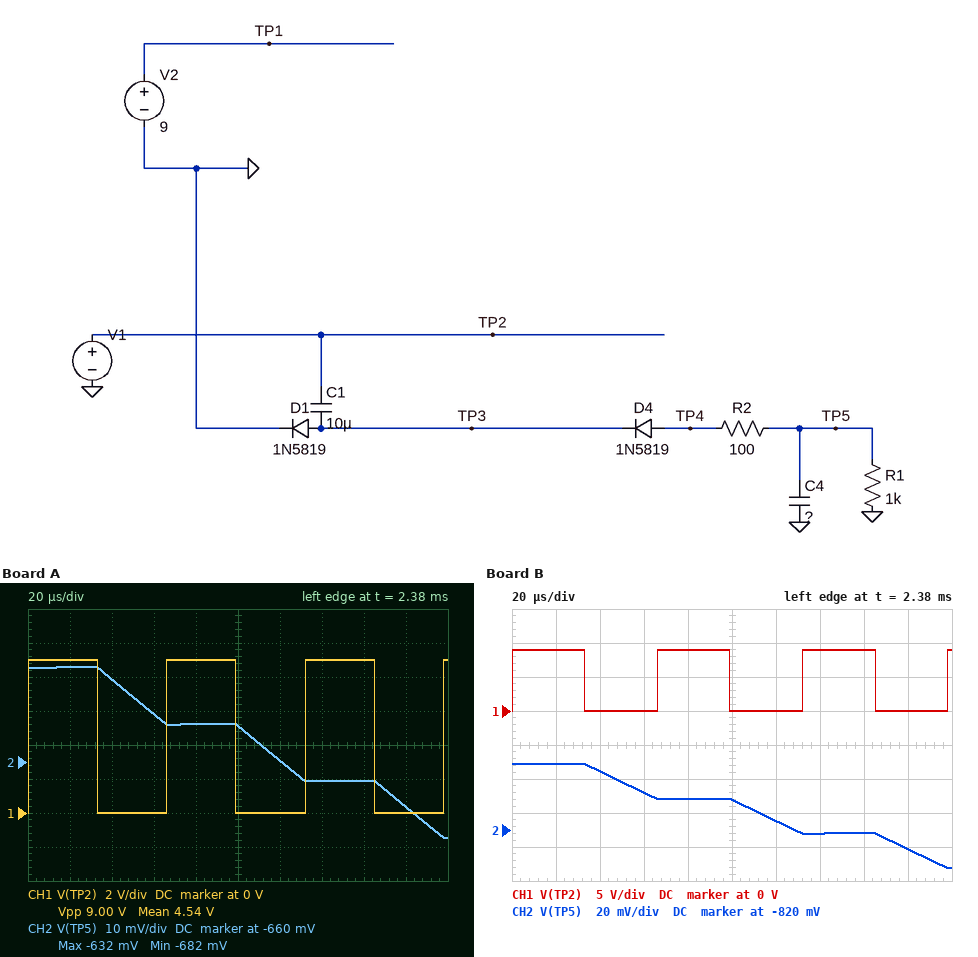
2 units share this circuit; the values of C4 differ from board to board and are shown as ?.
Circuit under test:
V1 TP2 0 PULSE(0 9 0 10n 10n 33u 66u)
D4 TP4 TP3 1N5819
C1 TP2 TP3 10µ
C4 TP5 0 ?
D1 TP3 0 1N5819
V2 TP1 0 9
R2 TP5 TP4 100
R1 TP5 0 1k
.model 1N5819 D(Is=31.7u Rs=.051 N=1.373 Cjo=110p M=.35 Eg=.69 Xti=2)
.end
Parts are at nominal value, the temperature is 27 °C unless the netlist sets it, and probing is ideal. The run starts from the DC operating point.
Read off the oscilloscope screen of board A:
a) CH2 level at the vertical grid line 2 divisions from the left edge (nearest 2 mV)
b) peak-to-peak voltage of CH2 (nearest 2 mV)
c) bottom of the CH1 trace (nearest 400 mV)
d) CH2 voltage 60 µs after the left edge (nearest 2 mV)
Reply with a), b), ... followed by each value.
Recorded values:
a) -636 mV
b) 50 mV
c) 0 V
d) -646 mV
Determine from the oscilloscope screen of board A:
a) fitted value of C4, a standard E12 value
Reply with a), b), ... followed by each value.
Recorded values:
a) 150 µF
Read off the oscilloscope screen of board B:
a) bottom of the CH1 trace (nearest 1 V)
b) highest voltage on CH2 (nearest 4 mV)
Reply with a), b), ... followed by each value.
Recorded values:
a) 0 V
b) -780 mV
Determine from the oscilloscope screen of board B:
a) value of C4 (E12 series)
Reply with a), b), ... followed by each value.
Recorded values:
a) 120 µF
